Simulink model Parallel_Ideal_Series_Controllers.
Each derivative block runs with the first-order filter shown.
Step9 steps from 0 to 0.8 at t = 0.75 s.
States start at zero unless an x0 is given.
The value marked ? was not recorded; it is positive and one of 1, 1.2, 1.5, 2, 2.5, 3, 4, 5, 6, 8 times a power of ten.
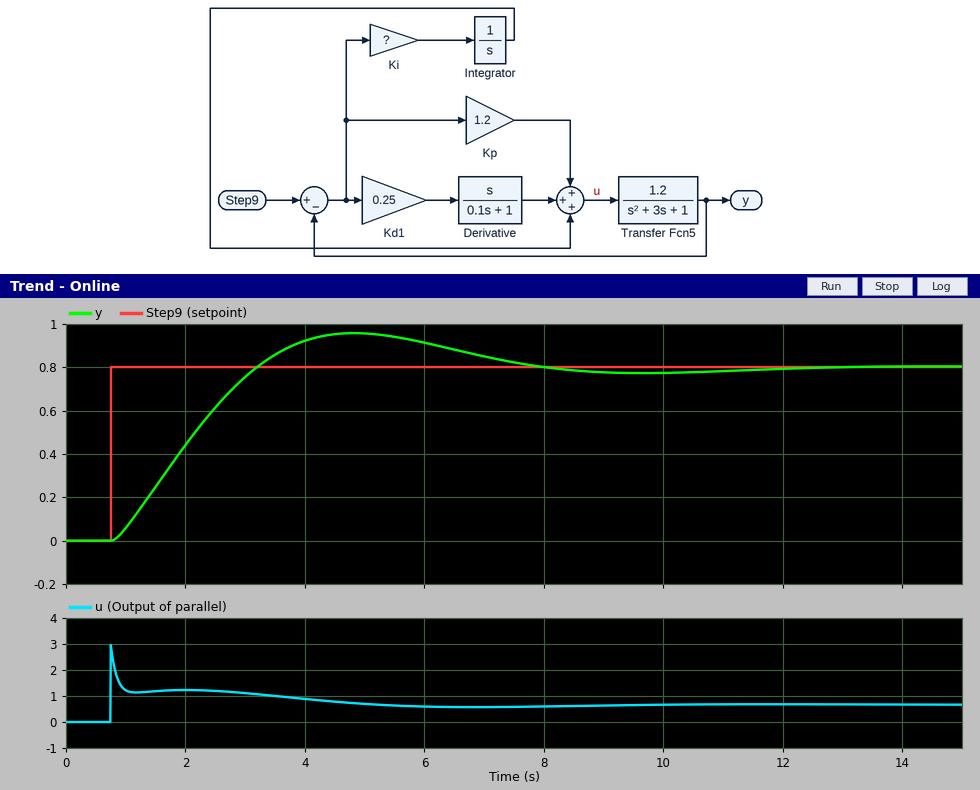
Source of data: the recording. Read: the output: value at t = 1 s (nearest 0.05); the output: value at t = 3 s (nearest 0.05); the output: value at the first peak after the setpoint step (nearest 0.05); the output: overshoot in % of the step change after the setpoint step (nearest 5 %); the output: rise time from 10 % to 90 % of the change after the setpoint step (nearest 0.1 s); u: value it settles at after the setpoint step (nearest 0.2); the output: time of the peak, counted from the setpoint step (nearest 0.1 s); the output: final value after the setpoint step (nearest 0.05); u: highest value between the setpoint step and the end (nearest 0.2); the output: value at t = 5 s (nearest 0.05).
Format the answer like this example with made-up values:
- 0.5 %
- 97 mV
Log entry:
- 0.05
- 0.75
- 0.95
- 20 %
- 1.8 s
- 0.6
- 4.1 s
- 0.80
- 3.0
- 0.95
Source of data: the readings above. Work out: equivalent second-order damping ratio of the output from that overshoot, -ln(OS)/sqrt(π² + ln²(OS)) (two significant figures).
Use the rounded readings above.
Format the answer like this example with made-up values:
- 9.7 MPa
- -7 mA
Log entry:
- 0.46
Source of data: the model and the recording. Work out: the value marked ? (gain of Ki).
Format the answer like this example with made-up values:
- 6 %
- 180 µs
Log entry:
- 1.2
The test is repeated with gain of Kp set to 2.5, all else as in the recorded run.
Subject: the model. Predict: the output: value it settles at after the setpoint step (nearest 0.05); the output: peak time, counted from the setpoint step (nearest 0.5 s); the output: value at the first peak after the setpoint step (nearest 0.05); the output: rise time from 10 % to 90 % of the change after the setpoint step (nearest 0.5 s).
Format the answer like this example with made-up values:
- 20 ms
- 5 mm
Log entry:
- 0.80
- 3.0 s
- 0.85
- 1.5 s
